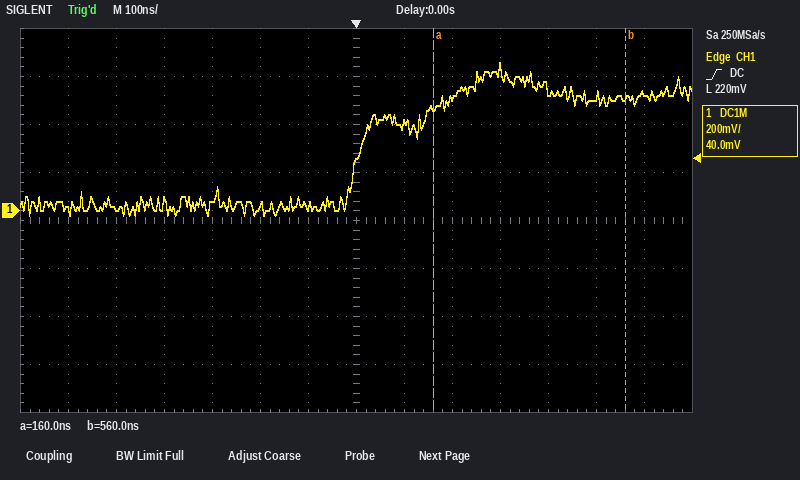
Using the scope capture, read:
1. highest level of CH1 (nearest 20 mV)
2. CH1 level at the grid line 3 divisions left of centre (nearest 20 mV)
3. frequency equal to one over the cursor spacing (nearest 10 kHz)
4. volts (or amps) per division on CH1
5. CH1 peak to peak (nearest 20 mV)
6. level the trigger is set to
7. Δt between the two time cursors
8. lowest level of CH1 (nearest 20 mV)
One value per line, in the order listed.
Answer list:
620 mV
40 mV
2.50 MHz
200 mV
640 mV
220 mV
400 ns
-20 mV
